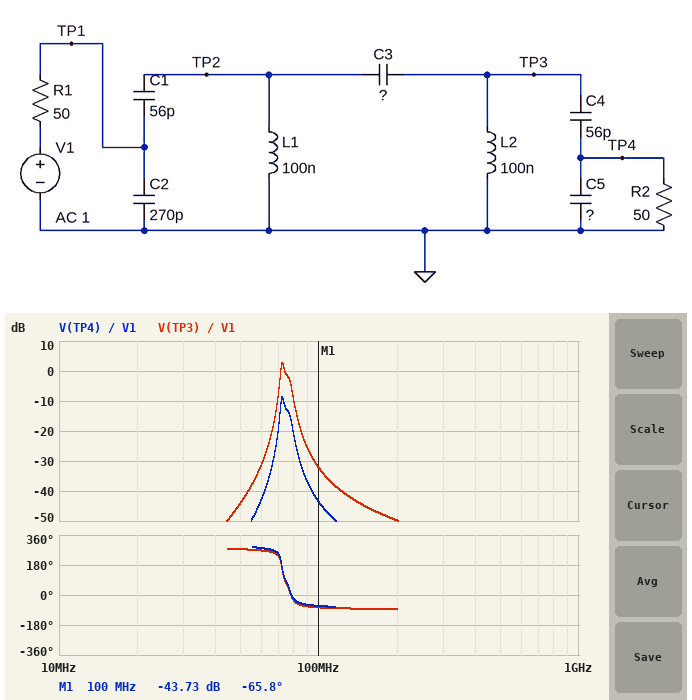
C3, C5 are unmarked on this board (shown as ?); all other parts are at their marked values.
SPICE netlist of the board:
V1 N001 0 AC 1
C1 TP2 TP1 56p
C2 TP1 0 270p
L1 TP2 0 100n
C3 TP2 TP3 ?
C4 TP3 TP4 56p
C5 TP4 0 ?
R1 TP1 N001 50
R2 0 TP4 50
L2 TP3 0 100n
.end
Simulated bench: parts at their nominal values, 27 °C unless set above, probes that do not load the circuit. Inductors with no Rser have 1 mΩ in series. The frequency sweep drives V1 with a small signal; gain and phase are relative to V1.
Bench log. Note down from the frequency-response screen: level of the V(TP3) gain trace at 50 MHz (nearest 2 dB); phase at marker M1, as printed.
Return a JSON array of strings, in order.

["-44 dB", "-65.8 deg"]
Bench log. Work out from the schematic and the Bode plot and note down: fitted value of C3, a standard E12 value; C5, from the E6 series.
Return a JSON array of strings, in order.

["1.8 pF", "150 pF"]
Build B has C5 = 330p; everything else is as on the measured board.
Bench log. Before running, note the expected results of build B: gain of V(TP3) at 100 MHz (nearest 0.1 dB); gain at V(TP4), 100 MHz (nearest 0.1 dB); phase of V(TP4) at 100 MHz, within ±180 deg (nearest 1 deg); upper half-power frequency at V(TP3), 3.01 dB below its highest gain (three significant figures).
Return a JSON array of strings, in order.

["-35.1 dB", "-51.9 dB", "-76 deg", "73.7 MHz"]
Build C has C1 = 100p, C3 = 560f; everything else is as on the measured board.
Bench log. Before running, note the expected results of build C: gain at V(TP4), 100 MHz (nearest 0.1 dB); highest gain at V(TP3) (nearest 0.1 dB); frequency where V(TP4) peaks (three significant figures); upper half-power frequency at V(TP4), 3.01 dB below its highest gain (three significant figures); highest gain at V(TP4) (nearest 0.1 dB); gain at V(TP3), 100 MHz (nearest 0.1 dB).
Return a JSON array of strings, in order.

["-55.9 dB", "-23.6 dB", "77.5 MHz", "80.1 MHz", "-35.1 dB", "-44.4 dB"]
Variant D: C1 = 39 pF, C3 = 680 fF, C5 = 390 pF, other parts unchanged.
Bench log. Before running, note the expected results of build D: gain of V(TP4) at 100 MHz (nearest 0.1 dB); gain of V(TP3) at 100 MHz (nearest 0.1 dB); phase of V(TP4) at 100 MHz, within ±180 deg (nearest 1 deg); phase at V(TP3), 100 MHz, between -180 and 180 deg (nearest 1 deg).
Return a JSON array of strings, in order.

["-56.6 dB", "-38.6 dB", "-76 deg", "-80 deg"]
